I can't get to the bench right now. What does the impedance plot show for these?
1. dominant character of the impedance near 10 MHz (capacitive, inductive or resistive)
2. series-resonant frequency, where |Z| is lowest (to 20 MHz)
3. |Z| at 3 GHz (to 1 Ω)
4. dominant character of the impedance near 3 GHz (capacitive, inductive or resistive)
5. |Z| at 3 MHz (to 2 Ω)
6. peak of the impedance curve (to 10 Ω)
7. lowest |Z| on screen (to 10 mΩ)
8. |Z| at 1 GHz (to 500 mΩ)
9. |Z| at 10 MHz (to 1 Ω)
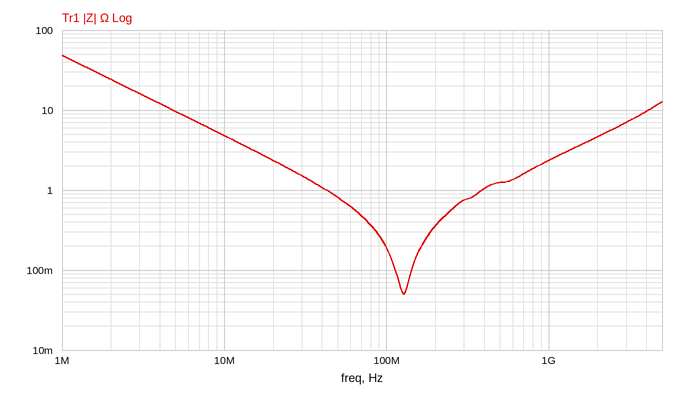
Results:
capacitive
120 MHz
7 Ω
inductive
16 Ω
50 Ω
50 mΩ
2.5 Ω
5 Ω
